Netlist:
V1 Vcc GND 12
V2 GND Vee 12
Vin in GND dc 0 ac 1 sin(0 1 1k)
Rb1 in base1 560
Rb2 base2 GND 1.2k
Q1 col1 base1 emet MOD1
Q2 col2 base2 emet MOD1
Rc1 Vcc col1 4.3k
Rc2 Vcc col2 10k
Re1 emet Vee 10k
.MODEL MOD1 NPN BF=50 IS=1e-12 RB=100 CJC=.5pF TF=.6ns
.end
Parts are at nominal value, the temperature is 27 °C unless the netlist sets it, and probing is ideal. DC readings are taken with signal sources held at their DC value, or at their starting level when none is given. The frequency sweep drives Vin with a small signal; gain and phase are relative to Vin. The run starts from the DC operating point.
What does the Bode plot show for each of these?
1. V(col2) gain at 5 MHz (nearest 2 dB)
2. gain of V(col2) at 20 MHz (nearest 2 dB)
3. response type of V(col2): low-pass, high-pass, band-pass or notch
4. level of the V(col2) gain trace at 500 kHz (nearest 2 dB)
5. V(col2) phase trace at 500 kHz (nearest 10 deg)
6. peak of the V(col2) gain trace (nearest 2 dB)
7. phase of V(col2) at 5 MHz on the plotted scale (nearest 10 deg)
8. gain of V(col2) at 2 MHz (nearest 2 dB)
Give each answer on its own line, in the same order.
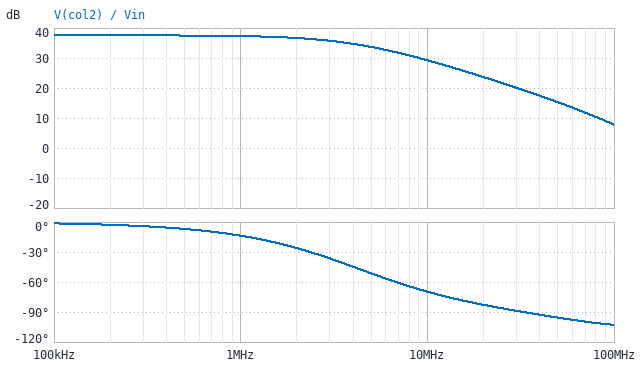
34 dB
24 dB
low-pass
38 dB
-10 deg
38 dB
-50 deg
36 dB
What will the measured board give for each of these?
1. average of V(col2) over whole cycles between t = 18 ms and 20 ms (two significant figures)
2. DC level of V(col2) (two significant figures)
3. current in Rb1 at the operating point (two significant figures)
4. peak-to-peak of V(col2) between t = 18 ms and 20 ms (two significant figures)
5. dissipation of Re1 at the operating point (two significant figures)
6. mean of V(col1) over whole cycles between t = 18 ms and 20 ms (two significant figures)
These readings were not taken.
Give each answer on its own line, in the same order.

6.4 V
6.9 V
12 µA
11 V
13 mW
9.4 V
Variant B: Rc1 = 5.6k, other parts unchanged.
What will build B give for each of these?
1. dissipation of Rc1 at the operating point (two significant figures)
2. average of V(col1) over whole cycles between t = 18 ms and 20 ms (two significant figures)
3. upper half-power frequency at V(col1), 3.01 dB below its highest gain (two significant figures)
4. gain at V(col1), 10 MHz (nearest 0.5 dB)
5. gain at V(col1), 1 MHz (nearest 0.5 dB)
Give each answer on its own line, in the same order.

2.1 mW
8.7 V
4.0 MHz
24.0 dB
32.5 dB
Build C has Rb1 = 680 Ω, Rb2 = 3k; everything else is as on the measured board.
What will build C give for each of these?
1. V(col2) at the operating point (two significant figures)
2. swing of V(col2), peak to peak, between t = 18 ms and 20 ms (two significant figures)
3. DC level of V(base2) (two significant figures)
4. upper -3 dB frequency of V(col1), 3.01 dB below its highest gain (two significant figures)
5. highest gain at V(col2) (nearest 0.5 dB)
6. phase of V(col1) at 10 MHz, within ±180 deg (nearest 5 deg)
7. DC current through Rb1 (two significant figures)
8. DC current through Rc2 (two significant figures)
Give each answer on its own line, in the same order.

7.9 V
11 V
-25 mV
2.7 MHz
35.0 dB
110 deg
14 µA
410 µA
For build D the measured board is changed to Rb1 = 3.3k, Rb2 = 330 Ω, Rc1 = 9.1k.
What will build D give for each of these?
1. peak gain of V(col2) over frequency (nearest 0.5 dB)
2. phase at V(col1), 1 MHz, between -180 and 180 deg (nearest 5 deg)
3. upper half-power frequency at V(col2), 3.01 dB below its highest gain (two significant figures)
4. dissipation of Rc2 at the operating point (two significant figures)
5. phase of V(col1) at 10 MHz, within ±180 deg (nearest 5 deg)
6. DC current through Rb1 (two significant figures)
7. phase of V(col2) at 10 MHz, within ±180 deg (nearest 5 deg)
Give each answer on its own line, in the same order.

35.0 dB
160 deg
2.7 MHz
5.7 mW
105 deg
7.4 µA
-80 deg
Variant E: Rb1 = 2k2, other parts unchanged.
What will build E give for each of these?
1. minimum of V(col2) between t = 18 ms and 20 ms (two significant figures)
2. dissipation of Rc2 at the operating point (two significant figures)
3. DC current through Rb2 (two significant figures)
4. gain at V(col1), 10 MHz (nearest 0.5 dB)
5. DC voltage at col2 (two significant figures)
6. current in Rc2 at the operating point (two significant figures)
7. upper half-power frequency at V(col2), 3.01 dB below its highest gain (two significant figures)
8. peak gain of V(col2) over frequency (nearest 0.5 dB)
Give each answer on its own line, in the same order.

790 mV
4.0 mW
13 µA
18.5 dB
5.7 V
630 µA
3.4 MHz
35.5 dB
